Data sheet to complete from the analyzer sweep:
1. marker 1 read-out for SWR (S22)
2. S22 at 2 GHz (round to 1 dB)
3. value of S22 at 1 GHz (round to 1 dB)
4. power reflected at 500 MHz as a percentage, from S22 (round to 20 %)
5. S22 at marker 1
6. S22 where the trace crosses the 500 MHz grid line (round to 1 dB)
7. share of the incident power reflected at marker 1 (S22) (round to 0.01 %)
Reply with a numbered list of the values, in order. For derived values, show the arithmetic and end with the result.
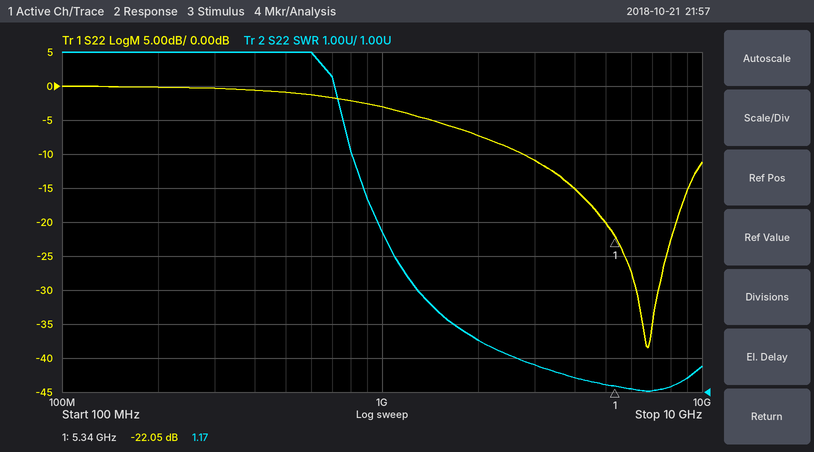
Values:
1. 1.17
2. -7 dB
3. -3 dB
4. 10^(-1/10) ≈ 79.4 %, so 80 % to the nearest 20 %
5. -22.05 dB
6. -1 dB
7. 10^(-22.05/10) ≈ 0.62 %
